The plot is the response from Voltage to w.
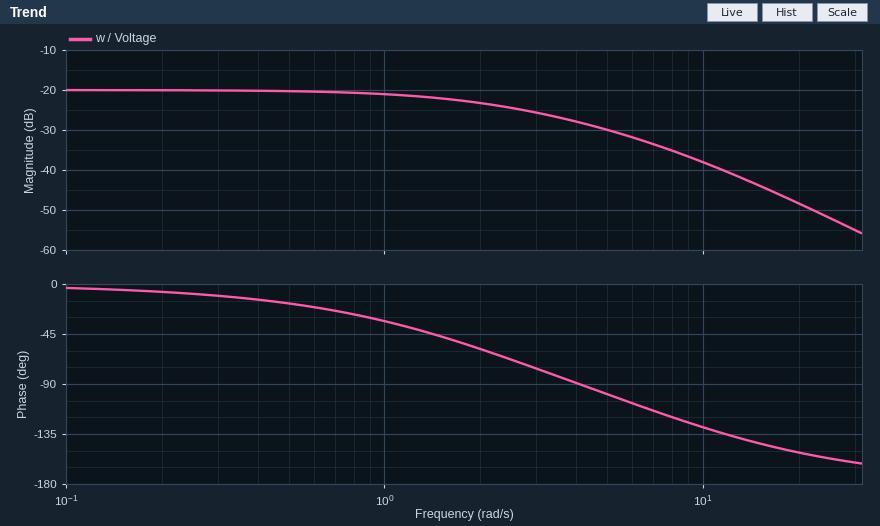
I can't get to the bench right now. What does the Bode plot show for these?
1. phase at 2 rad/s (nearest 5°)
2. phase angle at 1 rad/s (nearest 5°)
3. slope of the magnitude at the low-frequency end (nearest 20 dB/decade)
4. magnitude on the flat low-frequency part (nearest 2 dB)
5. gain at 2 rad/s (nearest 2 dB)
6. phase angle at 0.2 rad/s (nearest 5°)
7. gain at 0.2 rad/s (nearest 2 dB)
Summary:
-60°
-35°
0 dB/decade
-20 dB
-24 dB
-5°
-20 dB
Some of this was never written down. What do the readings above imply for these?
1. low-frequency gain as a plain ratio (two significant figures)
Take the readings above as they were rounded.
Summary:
0.10
